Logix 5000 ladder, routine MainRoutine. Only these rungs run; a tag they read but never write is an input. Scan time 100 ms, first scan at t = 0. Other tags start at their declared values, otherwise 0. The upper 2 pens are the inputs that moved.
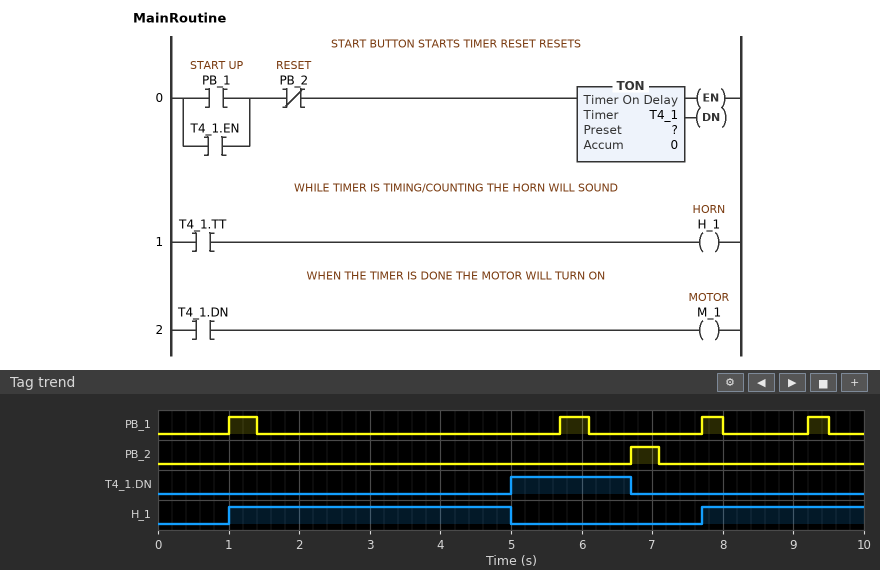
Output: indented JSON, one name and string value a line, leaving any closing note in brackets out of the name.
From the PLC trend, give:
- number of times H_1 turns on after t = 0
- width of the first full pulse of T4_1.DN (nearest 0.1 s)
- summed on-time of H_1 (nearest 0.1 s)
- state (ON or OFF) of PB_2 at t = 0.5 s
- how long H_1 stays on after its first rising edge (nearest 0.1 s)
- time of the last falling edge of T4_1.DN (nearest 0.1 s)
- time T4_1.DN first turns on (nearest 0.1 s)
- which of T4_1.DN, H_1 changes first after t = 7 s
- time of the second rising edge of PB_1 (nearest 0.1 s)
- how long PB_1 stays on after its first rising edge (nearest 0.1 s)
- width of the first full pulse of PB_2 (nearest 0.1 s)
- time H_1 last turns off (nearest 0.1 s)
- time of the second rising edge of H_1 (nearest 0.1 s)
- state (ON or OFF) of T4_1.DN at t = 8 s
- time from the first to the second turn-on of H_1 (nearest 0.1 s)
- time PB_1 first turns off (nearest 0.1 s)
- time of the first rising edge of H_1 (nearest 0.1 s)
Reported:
{
  "number of times H_1 turns on after t = 0": "2",
  "width of the first full pulse of T4_1.DN": "1.7 s",
  "summed on-time of H_1": "6.3 s",
  "state (ON or OFF) of PB_2 at t = 0.5 s": "OFF",
  "how long H_1 stays on after its first rising edge": "4.0 s",
  "time of the last falling edge of T4_1.DN": "6.7 s",
  "time T4_1.DN first turns on": "5.0 s",
  "which of T4_1.DN, H_1 changes first after t = 7 s": "H_1",
  "time of the second rising edge of PB_1": "5.7 s",
  "how long PB_1 stays on after its first rising edge": "0.4 s",
  "width of the first full pulse of PB_2": "0.4 s",
  "time H_1 last turns off": "5.0 s",
  "time of the second rising edge of H_1": "7.7 s",
  "state (ON or OFF) of T4_1.DN at t = 8 s": "OFF",
  "time from the first to the second turn-on of H_1": "6.7 s",
  "time PB_1 first turns off": "1.4 s",
  "time of the first rising edge of H_1": "1.0 s"
}
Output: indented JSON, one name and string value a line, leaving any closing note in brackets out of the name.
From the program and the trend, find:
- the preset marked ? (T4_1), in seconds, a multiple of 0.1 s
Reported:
{
  "the preset marked ? (T4_1), in seconds, a multiple of 0.1 s": "4.0 s"
}
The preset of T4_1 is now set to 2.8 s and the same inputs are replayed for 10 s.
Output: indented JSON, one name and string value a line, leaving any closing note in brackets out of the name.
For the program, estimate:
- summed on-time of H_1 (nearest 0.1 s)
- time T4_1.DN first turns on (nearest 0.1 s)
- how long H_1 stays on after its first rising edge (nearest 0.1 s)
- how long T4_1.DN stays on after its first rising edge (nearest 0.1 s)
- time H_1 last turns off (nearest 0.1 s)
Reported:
{
  "summed on-time of H_1": "5.1 s",
  "time T4_1.DN first turns on": "3.8 s",
  "how long H_1 stays on after its first rising edge": "2.8 s",
  "how long T4_1.DN stays on after its first rising edge": "2.9 s",
  "time H_1 last turns off": "3.8 s"
}
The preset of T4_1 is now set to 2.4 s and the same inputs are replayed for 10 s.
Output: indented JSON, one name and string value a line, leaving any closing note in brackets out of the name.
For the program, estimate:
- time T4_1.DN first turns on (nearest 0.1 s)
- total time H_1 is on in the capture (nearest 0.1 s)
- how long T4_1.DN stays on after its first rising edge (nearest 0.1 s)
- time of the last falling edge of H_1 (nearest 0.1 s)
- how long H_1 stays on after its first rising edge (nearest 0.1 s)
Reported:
{
  "time T4_1.DN first turns on": "3.4 s",
  "total time H_1 is on in the capture": "4.7 s",
  "how long T4_1.DN stays on after its first rising edge": "3.3 s",
  "time of the last falling edge of H_1": "3.4 s",
  "how long H_1 stays on after its first rising edge": "2.4 s"
}
